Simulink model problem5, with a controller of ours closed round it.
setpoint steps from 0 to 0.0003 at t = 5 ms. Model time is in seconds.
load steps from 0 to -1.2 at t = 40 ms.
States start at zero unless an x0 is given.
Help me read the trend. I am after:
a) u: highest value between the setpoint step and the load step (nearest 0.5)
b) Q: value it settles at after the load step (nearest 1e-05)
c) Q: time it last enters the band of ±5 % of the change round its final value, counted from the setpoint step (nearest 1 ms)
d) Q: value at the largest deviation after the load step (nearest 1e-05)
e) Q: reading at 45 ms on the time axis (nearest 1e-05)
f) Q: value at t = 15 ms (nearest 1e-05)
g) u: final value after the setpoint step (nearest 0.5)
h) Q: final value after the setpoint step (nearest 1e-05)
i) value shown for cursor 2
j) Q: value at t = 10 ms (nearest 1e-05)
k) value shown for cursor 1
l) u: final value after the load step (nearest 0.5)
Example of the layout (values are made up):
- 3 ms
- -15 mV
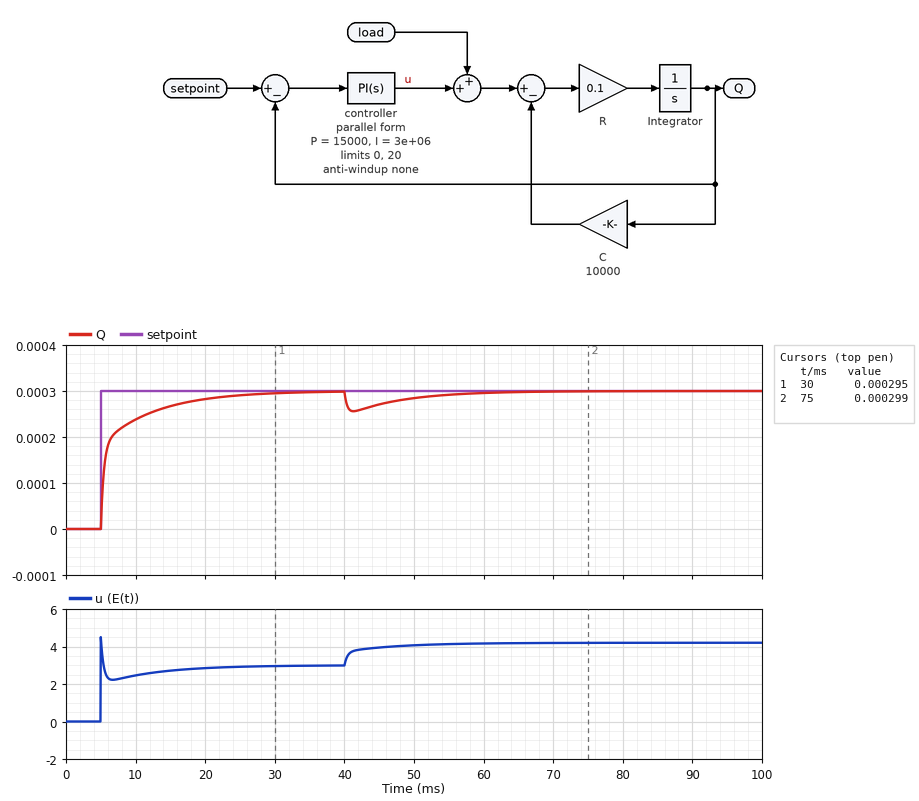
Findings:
- 4.5
- 0.00030
- 16 ms
- 0.00026
- 0.00027
- 0.00027
- 3.0
- 0.00030
- 0.000299
- 0.00024
- 0.000295
- 4.0
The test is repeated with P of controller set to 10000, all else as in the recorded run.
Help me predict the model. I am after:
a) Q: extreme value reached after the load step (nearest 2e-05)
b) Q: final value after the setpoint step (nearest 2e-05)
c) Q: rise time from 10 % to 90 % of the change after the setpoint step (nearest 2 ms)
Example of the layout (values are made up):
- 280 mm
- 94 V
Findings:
- 0.00024
- 0.00030
- 10 ms
